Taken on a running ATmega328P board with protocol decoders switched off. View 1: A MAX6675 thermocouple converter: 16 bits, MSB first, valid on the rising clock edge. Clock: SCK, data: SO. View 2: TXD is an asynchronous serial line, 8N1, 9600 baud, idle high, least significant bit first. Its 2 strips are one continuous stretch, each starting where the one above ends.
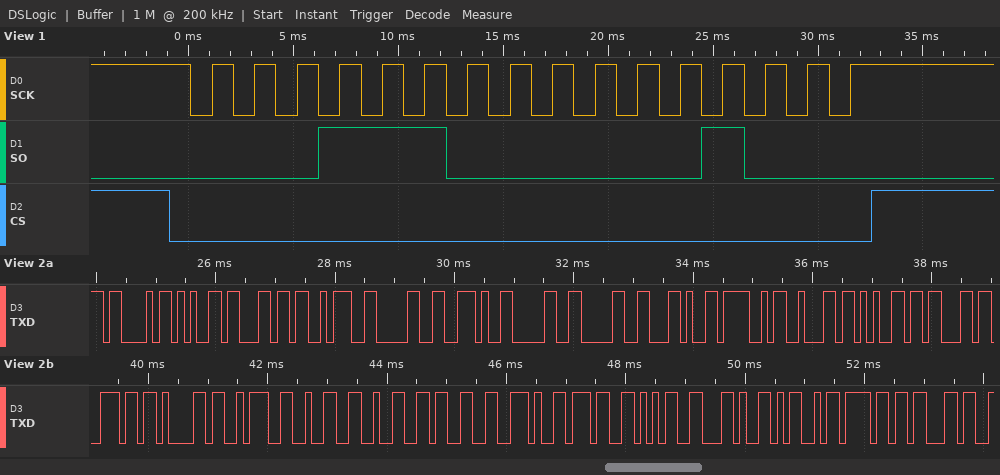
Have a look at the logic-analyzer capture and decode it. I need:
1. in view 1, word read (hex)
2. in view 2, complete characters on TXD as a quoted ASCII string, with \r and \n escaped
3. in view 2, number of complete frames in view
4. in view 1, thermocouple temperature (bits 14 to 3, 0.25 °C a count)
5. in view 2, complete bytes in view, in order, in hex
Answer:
0x1C08
"Cel:0.00,Obecna:223.75,Moc"
26
224.25 °C
43 65 6C 3A 30 2E 30 30 2C 4F 62 65 63 6E 61 3A 32 32 33 2E 37 35 2C 4D 6F 63
